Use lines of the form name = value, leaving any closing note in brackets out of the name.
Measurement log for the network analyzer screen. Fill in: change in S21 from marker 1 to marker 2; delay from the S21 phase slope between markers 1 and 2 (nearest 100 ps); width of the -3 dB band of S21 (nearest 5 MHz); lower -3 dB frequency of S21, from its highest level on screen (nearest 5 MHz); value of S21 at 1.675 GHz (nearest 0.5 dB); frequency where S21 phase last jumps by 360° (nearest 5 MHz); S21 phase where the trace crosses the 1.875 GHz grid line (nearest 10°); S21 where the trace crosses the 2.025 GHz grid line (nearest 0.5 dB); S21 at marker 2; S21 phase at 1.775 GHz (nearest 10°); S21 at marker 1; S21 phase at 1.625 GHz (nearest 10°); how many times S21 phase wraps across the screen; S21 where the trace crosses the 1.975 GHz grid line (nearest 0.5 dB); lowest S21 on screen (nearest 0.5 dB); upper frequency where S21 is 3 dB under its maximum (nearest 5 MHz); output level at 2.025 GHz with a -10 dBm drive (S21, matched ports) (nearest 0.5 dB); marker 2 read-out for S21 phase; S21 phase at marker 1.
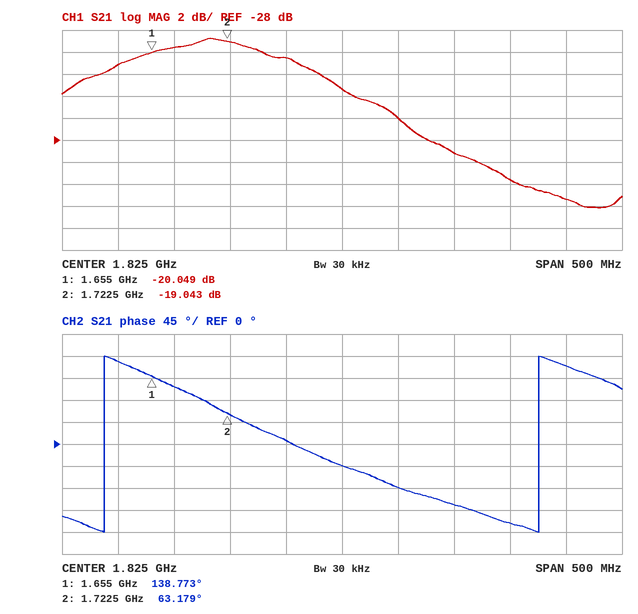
change in S21 from marker 1 to marker 2 = 1.006 dB
delay from the S21 phase slope between markers 1 and 2 = 3.1 ns
width of the -3 dB band of S21 = 185 MHz
lower -3 dB frequency of S21, from its highest level on screen = 1.615 GHz
value of S21 at 1.675 GHz = -19.5 dB
frequency where S21 phase last jumps by 360° = 2.000 GHz
S21 phase where the trace crosses the 1.875 GHz grid line = -90°
S21 where the trace crosses the 2.025 GHz grid line = -33.5 dB
S21 at marker 2 = -19.043 dB
S21 phase at 1.775 GHz = 10°
S21 at marker 1 = -20.049 dB
S21 phase at 1.625 GHz = 170°
how many times S21 phase wraps across the screen = 2
S21 where the trace crosses the 1.975 GHz grid line = -31.5 dB
lowest S21 on screen = -34.0 dB
upper frequency where S21 is 3 dB under its maximum = 1.800 GHz
output level at 2.025 GHz with a -10 dBm drive (S21, matched ports) = -43.5 dBm
marker 2 read-out for S21 phase = 63.179°
S21 phase at marker 1 = 138.773°
